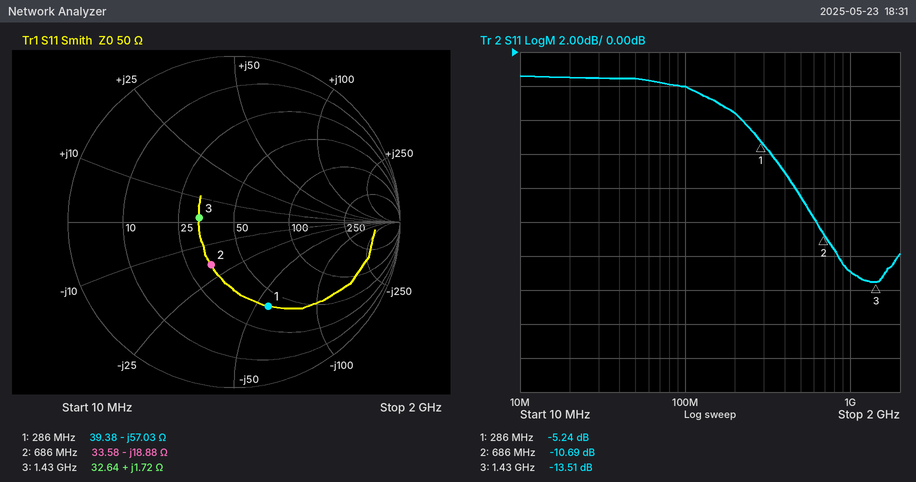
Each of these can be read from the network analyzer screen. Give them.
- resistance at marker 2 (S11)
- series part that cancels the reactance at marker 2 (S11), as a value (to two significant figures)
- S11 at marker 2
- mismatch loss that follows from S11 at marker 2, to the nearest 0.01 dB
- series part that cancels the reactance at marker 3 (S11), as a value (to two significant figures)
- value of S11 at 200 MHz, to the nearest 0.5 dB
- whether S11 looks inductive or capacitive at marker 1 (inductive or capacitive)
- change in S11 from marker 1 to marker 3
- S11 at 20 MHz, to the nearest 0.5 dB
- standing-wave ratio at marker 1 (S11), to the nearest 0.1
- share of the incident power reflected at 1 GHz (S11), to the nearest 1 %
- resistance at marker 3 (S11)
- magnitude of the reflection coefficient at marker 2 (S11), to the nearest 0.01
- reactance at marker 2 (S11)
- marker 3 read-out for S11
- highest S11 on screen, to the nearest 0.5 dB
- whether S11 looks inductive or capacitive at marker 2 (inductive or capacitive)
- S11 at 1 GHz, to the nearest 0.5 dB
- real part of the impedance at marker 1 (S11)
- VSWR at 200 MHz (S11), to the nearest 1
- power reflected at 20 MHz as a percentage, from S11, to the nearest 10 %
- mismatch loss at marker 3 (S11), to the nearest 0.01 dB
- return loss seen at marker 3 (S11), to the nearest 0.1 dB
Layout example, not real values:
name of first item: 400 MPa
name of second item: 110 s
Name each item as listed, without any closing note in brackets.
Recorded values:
resistance at marker 2: 33.58 Ω
series part that cancels the reactance at marker 2 (S11), as a value: 4.4 nH
S11 at marker 2: -10.69 dB
mismatch loss that follows from S11 at marker 2, to the nearest 0.01 dB: 0.39 dB
series part that cancels the reactance at marker 3 (S11), as a value: 65 pF
value of S11 at 200 MHz, to the nearest 0.5 dB: -3.5 dB
whether S11 looks inductive or capacitive at marker 1: capacitive
change in S11 from marker 1 to marker 3: -8.27 dB
S11 at 20 MHz, to the nearest 0.5 dB: -1.5 dB
standing-wave ratio at marker 1 (S11), to the nearest 0.1: 3.4
share of the incident power reflected at 1 GHz (S11), to the nearest 1 %: 5 %
resistance at marker 3: 32.64 Ω
magnitude of the reflection coefficient at marker 2 (S11), to the nearest 0.01: 0.29
reactance at marker 2: -18.88 Ω
marker 3 read-out for S11: -13.51 dB
highest S11 on screen, to the nearest 0.5 dB: -1.5 dB
whether S11 looks inductive or capacitive at marker 2: capacitive
S11 at 1 GHz, to the nearest 0.5 dB: -13.0 dB
real part of the impedance at marker 1: 39.38 Ω
VSWR at 200 MHz (S11), to the nearest 1: 5
power reflected at 20 MHz as a percentage, from S11, to the nearest 10 %: 70 %
mismatch loss at marker 3 (S11), to the nearest 0.01 dB: 0.20 dB
return loss seen at marker 3 (S11), to the nearest 0.1 dB: 13.5 dB
